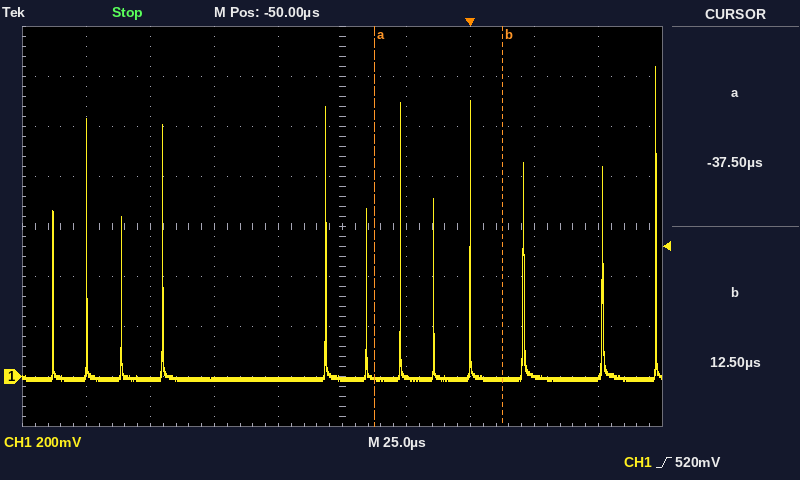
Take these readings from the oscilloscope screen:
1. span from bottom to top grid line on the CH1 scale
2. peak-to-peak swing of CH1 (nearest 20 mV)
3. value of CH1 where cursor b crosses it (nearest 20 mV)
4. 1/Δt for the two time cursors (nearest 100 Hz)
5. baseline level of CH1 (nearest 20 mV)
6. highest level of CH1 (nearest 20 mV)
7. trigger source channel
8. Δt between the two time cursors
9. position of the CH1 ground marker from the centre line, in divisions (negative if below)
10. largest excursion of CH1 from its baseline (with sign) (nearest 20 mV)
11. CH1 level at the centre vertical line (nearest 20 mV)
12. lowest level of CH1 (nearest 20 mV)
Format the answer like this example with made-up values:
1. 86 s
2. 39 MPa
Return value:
1. 1.6 V
2. 1.26 V
3. -20 mV
4. 20.0 kHz
5. -20 mV
6. 1.24 V
7. CH1
8. 50.0 µs
9. -3.0 div
10. +1.26 V
11. -20 mV
12. -20 mV
